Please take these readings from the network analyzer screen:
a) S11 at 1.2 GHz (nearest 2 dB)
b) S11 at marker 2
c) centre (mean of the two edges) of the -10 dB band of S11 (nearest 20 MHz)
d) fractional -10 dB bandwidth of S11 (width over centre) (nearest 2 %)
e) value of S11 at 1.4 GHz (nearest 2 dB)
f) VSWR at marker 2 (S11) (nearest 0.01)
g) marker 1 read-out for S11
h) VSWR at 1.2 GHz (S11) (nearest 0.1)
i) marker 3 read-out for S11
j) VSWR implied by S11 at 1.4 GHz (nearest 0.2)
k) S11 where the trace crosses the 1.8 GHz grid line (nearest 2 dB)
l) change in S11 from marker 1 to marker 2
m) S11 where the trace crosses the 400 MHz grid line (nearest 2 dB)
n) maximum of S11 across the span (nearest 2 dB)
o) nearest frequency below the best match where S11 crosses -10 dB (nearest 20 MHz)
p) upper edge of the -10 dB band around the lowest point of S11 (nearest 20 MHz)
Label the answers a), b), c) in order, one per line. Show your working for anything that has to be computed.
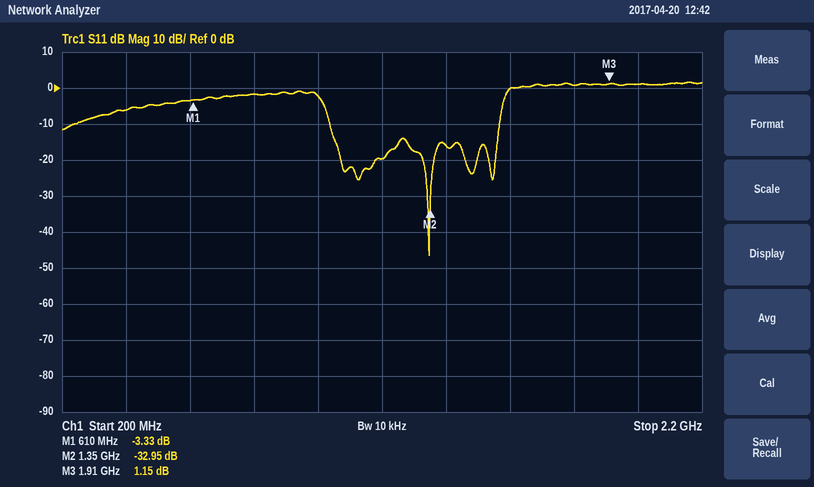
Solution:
a) -20 dB
b) -32.95 dB
c) 1.30 GHz
d) 520 MHz / 1.3 GHz ≈ 40 %
e) -16 dB
f) (1 + 0.0225)/(1 − 0.0225) ≈ 1.05
g) -3.33 dB
h) |Γ| = 10^(-20/20) = 0.1000; VSWR = (1 + 0.1000)/(1 − 0.1000) ≈ 1.2
i) 1.15 dB
j) |Γ| = 10^(-16/20) = 0.1585; VSWR = (1 + 0.1585)/(1 − 0.1585) ≈ 1.4
k) 0 dB
l) -32.95 − (-3.33) = -29.62 dB
m) -6 dB
n) 2 dB
o) 1.04 GHz
p) 1.56 GHz
